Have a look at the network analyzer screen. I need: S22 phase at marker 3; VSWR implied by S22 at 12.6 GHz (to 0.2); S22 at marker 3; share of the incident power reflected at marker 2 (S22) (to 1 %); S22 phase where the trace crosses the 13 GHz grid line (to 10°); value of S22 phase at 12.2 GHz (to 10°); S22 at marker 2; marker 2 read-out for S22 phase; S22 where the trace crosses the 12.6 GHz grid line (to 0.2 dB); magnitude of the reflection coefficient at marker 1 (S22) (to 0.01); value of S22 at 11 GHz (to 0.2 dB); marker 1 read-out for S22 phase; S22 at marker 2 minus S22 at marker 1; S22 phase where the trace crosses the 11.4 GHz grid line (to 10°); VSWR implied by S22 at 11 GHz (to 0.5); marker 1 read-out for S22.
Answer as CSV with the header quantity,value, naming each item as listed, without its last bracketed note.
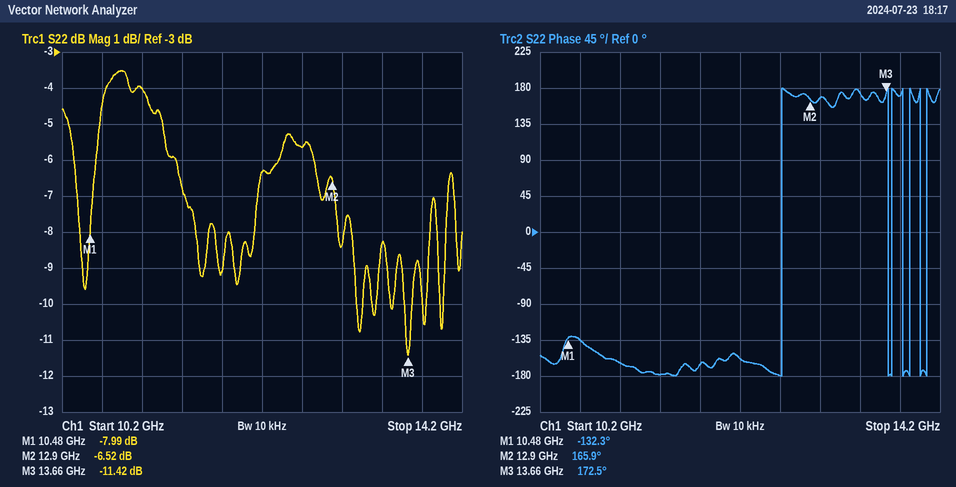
quantity,value
S22 phase at marker 3,172.5°
VSWR implied by S22 at 12.6 GHz,3.2
S22 at marker 3,-11.42 dB
share of the incident power reflected at marker 2 (S22),22 %
S22 phase where the trace crosses the 13 GHz grid line,170°
value of S22 phase at 12.2 GHz,-160°
S22 at marker 2,-6.52 dB
marker 2 read-out for S22 phase,165.9°
S22 where the trace crosses the 12.6 GHz grid line,-5.6 dB
magnitude of the reflection coefficient at marker 1 (S22),0.40
value of S22 at 11 GHz,-4.0 dB
marker 1 read-out for S22 phase,-132.3°
S22 at marker 2 minus S22 at marker 1,1.47 dB
S22 phase where the trace crosses the 11.4 GHz grid line,-180°
VSWR implied by S22 at 11 GHz,4.5
marker 1 read-out for S22,-7.99 dB
